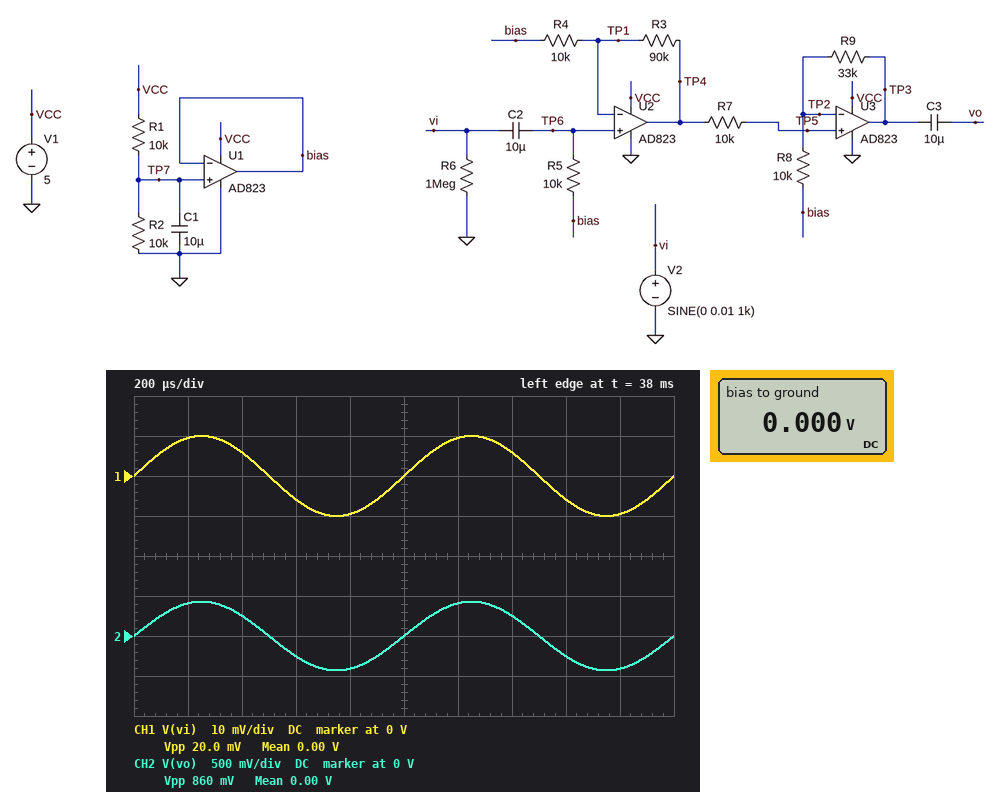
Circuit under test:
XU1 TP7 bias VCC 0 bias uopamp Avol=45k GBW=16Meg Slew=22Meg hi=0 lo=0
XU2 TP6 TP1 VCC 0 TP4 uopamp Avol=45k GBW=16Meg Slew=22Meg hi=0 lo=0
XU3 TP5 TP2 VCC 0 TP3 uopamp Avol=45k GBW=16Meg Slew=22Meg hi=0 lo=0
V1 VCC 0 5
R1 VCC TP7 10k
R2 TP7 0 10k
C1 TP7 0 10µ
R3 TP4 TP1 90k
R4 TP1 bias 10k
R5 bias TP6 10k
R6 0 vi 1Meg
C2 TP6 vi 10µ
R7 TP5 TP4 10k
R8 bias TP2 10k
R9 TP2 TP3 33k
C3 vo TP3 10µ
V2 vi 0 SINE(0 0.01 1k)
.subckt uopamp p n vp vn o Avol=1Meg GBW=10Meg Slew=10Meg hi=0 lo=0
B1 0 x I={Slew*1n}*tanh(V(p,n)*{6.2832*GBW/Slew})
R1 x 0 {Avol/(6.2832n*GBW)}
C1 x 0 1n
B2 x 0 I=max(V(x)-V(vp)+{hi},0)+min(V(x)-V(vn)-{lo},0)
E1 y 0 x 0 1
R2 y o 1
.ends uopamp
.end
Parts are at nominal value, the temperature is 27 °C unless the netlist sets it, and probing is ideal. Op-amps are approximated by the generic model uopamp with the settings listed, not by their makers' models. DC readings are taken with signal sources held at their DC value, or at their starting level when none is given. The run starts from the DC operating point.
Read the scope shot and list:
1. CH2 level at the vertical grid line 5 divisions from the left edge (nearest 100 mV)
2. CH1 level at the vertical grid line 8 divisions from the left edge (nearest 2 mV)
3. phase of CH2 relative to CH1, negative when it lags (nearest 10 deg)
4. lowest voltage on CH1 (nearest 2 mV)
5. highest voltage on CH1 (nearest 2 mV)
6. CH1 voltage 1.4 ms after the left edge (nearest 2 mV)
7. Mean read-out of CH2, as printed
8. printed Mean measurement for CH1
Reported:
0 V
-6 mV
0 deg
-10 mV
10 mV
6 mV
0.00 V
0.00 V
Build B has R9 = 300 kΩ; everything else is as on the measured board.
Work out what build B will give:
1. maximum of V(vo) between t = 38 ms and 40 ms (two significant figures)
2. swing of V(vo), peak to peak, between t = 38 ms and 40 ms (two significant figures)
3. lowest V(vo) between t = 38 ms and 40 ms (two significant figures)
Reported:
2.5 V
5.0 V
-2.5 V
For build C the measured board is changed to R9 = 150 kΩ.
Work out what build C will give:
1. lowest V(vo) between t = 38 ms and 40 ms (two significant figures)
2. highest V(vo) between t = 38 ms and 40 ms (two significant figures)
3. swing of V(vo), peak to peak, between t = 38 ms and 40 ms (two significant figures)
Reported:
-1.6 V
1.6 V
3.2 V
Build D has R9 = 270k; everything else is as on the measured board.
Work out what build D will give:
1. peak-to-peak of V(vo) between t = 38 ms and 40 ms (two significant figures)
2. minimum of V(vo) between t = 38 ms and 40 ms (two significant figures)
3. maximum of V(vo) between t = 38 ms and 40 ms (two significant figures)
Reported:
5.0 V
-2.5 V
2.5 V
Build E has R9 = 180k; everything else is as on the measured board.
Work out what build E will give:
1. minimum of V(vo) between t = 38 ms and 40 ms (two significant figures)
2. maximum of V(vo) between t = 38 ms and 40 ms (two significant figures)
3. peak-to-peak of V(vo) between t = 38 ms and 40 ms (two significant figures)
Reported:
-1.9 V
1.9 V
3.8 V
